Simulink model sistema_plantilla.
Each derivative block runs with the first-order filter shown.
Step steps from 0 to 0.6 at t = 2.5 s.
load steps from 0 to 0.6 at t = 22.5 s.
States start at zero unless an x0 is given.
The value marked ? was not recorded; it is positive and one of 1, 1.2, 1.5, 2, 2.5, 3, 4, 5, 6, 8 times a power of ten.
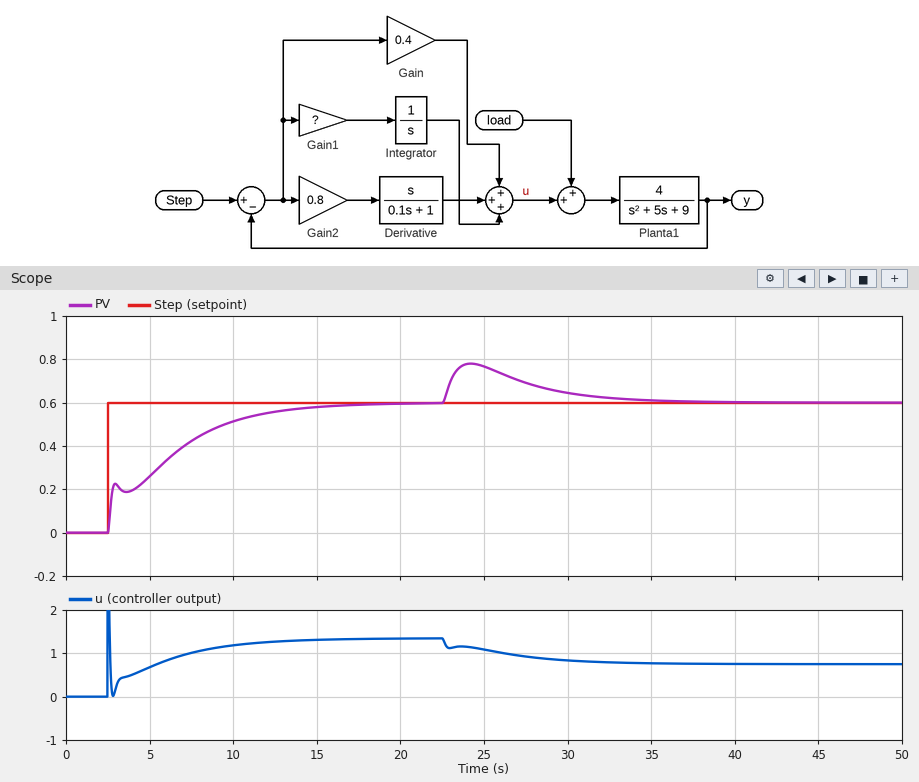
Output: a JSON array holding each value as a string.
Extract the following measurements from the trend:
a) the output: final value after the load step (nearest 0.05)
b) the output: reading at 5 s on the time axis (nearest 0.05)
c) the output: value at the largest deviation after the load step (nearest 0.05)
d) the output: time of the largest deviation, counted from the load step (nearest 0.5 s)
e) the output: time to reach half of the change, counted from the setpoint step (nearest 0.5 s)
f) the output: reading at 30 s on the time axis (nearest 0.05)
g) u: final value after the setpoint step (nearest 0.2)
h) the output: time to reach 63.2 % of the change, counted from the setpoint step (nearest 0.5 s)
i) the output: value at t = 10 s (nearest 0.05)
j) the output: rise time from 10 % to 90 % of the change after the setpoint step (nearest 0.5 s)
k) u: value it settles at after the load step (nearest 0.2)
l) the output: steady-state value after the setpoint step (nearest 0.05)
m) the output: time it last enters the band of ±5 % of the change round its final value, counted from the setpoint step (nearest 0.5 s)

["0.60", "0.25", "0.80", "1.5 s", "3.0 s", "0.65", "1.4", "4.0 s", "0.50", "8.5 s", "0.8", "0.60", "11.0 s"]
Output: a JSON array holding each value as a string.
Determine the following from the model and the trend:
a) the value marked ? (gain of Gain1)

["0.6"]
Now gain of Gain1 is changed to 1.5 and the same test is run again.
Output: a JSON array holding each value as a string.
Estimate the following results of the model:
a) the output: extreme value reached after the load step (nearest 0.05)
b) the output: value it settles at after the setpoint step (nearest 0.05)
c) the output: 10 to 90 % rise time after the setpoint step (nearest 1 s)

["0.75", "0.60", "3 s"]
